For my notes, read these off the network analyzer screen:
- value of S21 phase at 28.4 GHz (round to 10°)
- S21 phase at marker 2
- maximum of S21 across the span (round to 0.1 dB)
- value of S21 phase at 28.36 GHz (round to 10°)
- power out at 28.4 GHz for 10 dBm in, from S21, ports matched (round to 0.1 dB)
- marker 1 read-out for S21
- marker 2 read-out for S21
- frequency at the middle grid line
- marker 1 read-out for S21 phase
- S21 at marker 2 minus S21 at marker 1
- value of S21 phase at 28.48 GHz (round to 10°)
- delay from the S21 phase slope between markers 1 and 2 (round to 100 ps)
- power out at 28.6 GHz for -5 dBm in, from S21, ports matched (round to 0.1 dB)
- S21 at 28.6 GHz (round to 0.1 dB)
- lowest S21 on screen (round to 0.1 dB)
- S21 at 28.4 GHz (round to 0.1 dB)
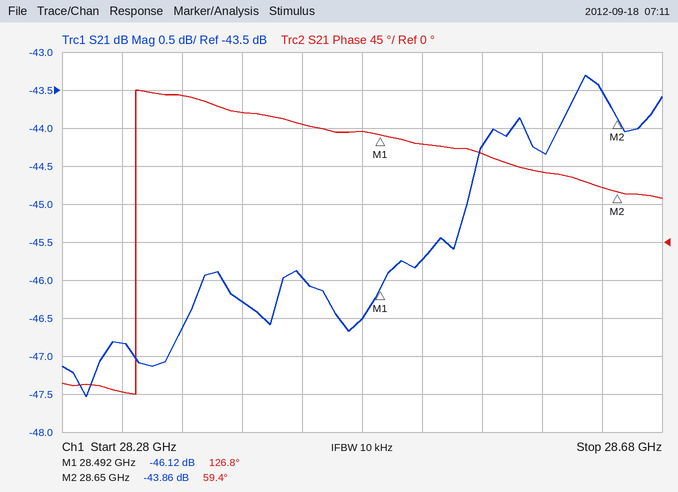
150°
59.4°
-43.3 dB
170°
-36.3 dBm
-46.12 dB
-43.86 dB
28.48 GHz
126.8°
2.26 dB
130°
1.2 ns
-49.3 dBm
-44.3 dB
-47.5 dB
-46.3 dB
